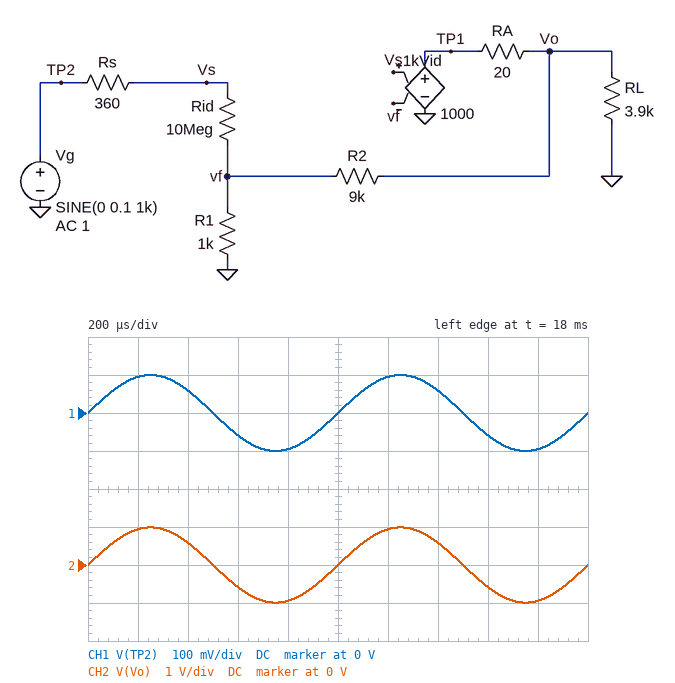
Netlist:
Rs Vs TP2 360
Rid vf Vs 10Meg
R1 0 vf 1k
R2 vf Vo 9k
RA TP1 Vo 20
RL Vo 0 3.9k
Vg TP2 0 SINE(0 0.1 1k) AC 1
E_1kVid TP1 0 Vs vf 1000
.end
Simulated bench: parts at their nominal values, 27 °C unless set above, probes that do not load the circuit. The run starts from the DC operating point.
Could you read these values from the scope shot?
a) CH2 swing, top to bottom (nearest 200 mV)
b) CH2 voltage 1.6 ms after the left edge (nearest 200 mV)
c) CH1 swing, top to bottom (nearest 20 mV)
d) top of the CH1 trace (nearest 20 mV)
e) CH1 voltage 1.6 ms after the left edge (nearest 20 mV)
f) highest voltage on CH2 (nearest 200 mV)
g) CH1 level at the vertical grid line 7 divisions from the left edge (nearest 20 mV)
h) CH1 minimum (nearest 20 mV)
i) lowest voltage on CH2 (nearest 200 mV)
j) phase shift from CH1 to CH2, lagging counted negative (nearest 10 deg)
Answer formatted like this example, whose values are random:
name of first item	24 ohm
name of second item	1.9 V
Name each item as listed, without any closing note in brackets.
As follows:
CH2 swing, top to bottom	2.0 V
CH2 voltage 1.6 ms after the left edge	-600 mV
CH1 swing, top to bottom	200 mV
top of the CH1 trace	100 mV
CH1 voltage 1.6 ms after the left edge	-60 mV
highest voltage on CH2	1.0 V
CH1 level at the vertical grid line 7 divisions from the left edge	60 mV
CH1 minimum	-100 mV
lowest voltage on CH2	-1.0 V
phase shift from CH1 to CH2, lagging counted negative	0 deg
